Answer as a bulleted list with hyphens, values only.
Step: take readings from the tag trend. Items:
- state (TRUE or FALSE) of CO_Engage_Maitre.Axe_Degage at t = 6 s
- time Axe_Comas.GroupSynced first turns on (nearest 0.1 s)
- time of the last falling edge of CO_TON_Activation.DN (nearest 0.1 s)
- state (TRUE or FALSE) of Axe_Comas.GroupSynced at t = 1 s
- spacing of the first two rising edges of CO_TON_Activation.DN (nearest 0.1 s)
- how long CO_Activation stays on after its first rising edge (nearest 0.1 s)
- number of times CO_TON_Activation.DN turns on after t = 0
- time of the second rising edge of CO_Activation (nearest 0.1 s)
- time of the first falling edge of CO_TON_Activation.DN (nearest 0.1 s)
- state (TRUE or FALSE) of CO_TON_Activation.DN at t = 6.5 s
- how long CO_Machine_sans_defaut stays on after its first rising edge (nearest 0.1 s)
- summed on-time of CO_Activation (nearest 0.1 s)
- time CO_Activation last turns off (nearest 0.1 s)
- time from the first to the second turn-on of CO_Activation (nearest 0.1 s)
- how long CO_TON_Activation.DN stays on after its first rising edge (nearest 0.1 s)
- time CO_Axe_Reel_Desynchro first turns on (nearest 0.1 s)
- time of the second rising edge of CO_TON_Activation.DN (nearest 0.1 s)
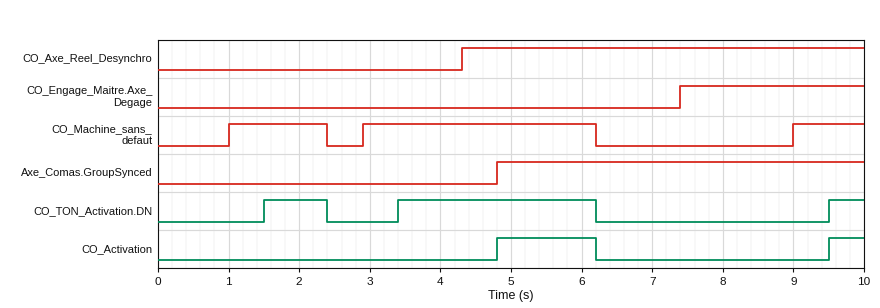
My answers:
- FALSE
- 4.8 s
- 6.2 s
- FALSE
- 1.9 s
- 1.4 s
- 3
- 9.5 s
- 2.4 s
- FALSE
- 1.4 s
- 1.9 s
- 6.2 s
- 4.7 s
- 0.9 s
- 4.3 s
- 3.4 s
